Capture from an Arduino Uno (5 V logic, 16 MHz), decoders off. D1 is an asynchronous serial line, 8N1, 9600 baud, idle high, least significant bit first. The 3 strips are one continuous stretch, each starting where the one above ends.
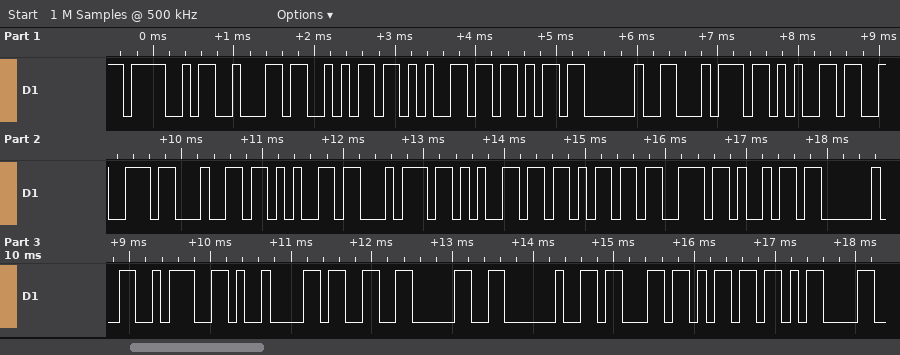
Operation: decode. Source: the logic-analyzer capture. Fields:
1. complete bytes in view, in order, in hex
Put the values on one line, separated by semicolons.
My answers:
4F 62 6A 65 6B 20 74 65 72 64 65 74 65 6B 73 69 20 3A 09 33 30 20 63 6D 0D
